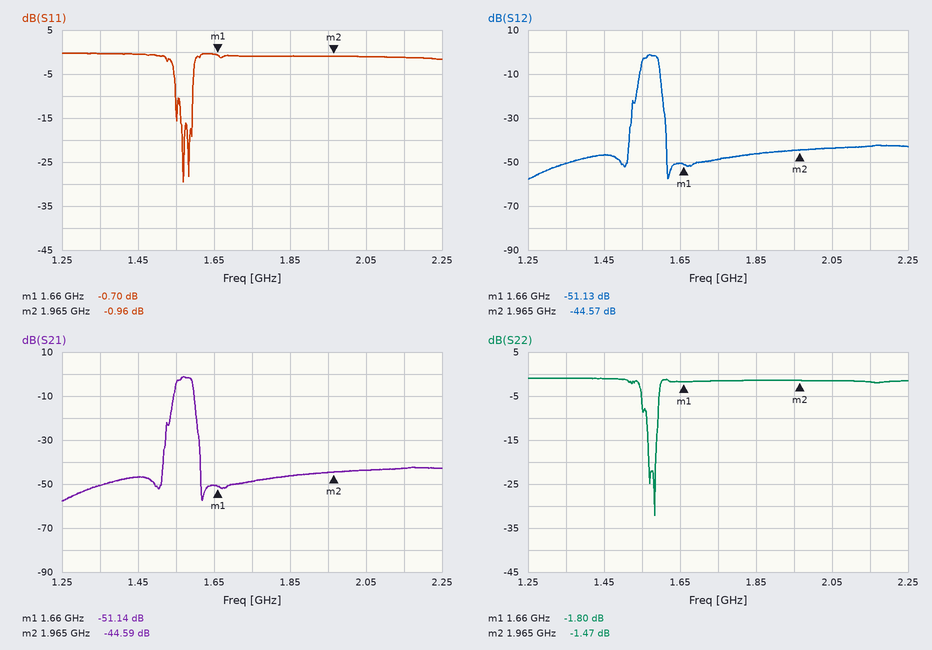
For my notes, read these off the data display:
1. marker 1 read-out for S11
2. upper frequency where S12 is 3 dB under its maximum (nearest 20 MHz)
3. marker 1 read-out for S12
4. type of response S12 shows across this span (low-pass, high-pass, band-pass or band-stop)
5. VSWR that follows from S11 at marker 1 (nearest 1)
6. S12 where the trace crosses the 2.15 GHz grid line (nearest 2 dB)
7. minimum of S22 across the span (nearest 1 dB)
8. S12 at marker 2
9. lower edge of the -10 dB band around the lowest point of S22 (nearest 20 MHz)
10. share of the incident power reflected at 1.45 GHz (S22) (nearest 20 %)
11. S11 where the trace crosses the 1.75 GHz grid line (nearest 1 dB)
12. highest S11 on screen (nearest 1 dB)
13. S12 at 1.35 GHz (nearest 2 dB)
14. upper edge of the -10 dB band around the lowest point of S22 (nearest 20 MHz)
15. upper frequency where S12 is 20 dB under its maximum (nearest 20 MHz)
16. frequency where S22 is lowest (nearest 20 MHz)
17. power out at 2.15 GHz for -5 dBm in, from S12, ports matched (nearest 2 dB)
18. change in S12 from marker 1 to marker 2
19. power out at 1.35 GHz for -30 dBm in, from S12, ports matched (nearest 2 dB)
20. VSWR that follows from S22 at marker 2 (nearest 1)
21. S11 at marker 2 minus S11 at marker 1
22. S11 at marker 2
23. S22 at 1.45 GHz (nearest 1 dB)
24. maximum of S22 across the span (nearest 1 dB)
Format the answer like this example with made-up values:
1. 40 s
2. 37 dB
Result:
1. -0.70 dB
2. 1.60 GHz
3. -51.13 dB
4. band-pass
5. 25
6. -42 dB
7. -32 dB
8. -44.57 dB
9. 1.56 GHz
10. 80 %
11. -1 dB
12. 0 dB
13. -50 dB
14. 1.60 GHz
15. 1.60 GHz
16. 1.58 GHz
17. -48 dBm
18. 6.56 dB
19. -80 dBm
20. 12
21. -0.26 dB
22. -0.96 dB
23. -1 dB
24. -1 dB
